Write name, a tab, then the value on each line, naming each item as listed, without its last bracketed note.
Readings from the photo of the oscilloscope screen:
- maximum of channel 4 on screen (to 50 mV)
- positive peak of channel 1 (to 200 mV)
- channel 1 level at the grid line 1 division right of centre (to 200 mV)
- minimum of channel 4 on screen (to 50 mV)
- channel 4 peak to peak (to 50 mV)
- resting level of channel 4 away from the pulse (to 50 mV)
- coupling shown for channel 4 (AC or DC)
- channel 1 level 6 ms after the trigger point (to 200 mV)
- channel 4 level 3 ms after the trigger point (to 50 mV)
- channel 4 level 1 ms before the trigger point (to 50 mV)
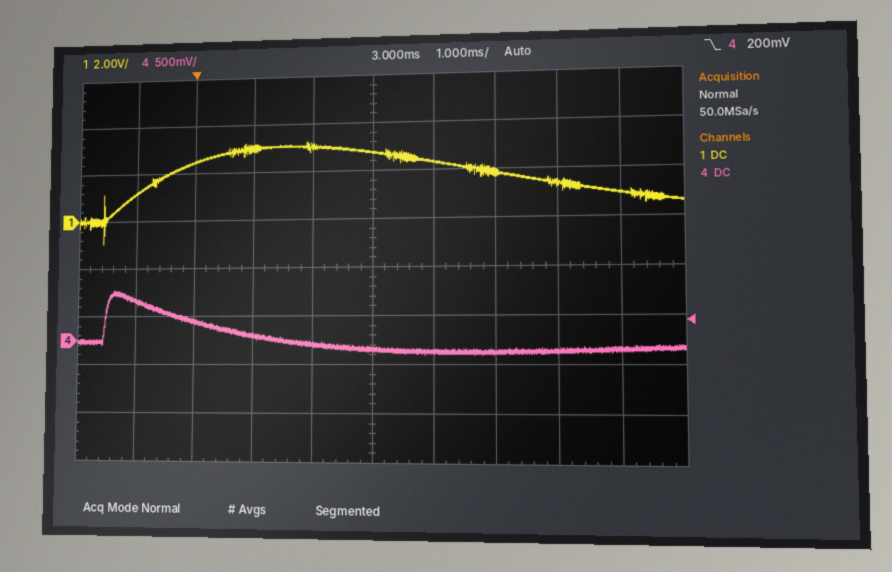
maximum of channel 4 on screen	500 mV
positive peak of channel 1	3.2 V
channel 1 level at the grid line 1 division right of centre	2.4 V
minimum of channel 4 on screen	-150 mV
channel 4 peak to peak	650 mV
resting level of channel 4 away from the pulse	-100 mV
coupling shown for channel 4	DC
channel 1 level 6 ms after the trigger point	1.4 V
channel 4 level 3 ms after the trigger point	-100 mV
channel 4 level 1 ms before the trigger point	400 mV
